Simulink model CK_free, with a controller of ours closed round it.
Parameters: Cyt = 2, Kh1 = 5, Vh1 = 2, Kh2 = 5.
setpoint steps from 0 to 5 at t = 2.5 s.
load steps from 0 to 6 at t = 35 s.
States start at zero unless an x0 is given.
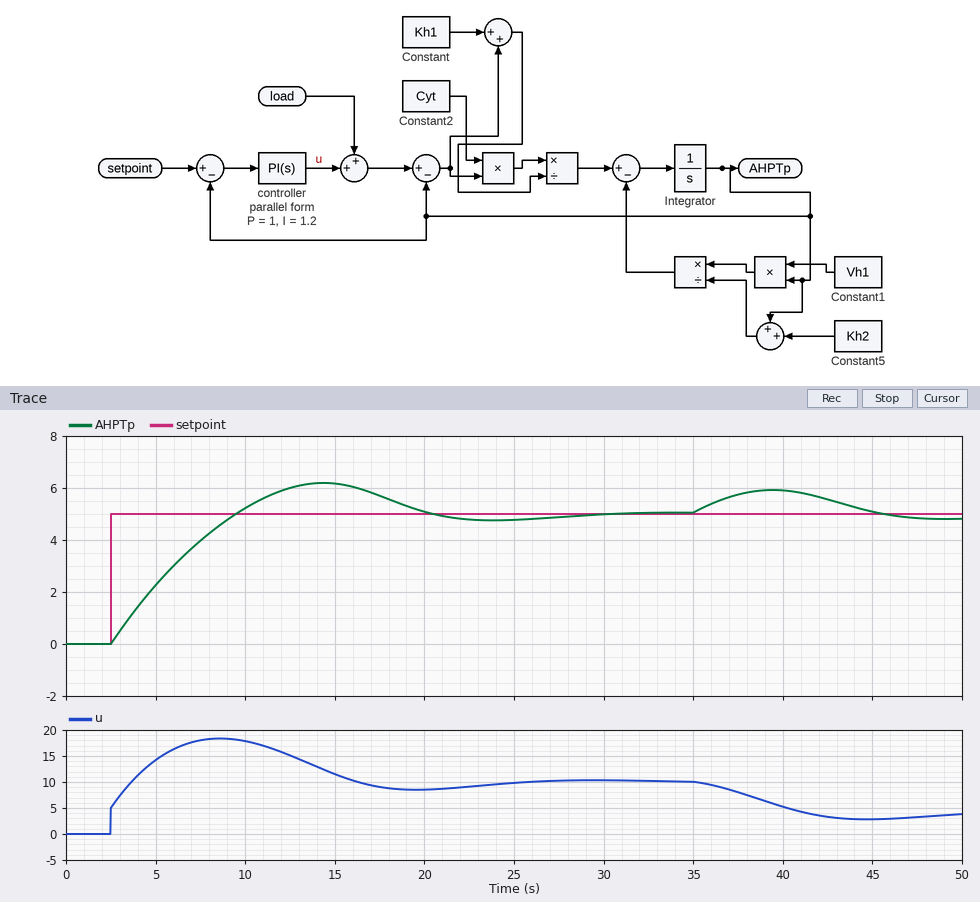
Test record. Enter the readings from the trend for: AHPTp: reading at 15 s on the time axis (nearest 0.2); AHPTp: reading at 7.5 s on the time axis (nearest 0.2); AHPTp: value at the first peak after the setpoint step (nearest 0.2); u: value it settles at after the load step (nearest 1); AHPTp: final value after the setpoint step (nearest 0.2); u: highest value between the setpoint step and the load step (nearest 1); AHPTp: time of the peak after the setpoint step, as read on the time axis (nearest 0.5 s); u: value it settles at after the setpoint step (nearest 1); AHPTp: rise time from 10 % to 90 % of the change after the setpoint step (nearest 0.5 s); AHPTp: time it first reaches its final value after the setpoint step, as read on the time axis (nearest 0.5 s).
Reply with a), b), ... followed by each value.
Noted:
a) 6.2
b) 4.0
c) 6.2
d) 4
e) 5.0
f) 18
g) 14.5 s
h) 10
i) 5.5 s
j) 9.5 s
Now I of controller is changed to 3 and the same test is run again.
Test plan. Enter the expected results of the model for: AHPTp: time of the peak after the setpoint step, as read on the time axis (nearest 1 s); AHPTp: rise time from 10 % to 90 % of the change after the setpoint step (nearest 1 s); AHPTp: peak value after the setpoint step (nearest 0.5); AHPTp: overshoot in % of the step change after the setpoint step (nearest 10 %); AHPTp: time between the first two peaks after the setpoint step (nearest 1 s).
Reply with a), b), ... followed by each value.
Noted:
a) 12 s
b) 4 s
c) 7.0
d) 40 %
e) 11 s
